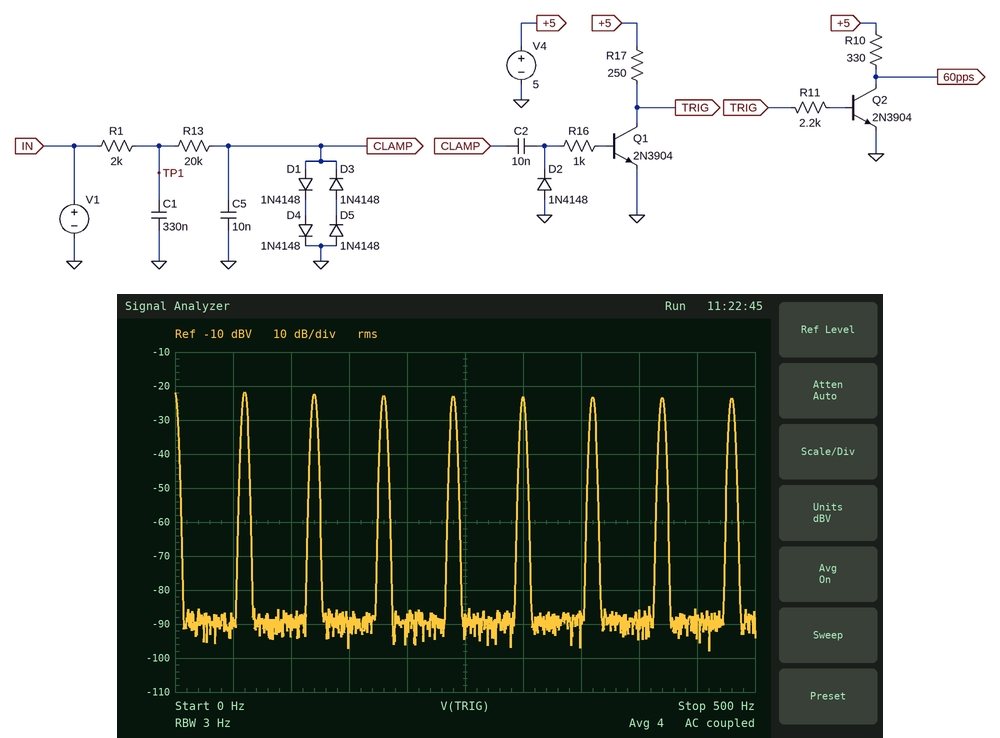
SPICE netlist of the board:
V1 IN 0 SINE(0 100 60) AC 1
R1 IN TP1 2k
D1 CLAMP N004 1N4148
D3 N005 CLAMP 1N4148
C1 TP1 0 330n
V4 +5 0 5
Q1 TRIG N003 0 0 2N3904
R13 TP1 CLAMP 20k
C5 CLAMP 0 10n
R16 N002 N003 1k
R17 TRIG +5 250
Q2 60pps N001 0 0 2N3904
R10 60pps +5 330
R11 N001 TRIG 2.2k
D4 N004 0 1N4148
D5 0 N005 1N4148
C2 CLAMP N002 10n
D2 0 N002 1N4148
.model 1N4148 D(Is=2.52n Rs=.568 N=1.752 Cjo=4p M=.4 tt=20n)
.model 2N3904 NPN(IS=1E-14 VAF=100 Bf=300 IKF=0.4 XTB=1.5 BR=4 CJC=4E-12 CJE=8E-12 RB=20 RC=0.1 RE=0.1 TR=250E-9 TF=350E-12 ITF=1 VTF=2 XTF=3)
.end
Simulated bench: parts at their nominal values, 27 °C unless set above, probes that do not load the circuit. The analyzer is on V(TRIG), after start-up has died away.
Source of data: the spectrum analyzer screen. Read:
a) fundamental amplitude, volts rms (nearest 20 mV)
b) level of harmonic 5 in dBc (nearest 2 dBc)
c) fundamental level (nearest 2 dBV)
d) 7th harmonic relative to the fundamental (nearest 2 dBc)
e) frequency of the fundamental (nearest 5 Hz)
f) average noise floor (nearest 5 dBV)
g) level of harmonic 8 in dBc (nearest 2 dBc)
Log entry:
80 mV
-2 dBc
-22 dBV
-2 dBc
60 Hz
-90 dBV
-2 dBc
